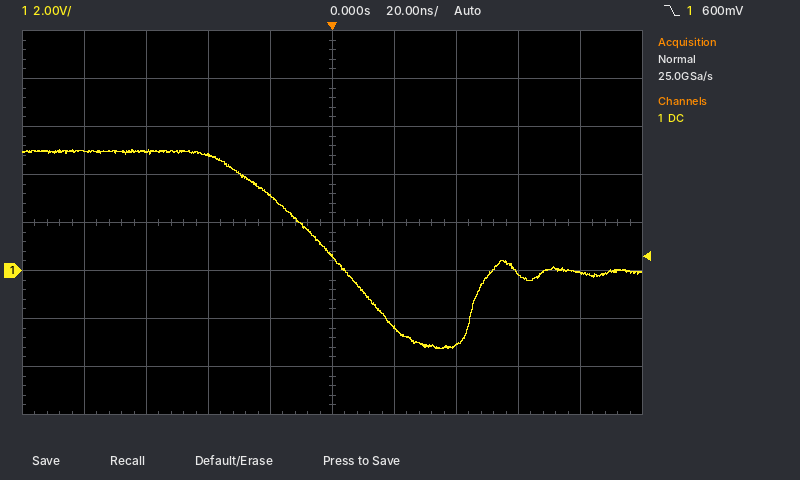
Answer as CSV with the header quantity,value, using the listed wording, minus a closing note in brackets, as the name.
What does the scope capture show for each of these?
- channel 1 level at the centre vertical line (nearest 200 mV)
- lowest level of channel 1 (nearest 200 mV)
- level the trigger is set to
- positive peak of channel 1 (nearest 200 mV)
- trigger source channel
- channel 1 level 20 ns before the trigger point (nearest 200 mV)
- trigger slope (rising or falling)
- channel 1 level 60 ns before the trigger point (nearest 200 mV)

quantity,value
channel 1 level at the centre vertical line,600 mV
lowest level of channel 1,-3.2 V
level the trigger is set to,600 mV
positive peak of channel 1,5.0 V
trigger source channel,channel 1
channel 1 level 20 ns before the trigger point,3.2 V
trigger slope,falling
channel 1 level 60 ns before the trigger point,5.0 V
